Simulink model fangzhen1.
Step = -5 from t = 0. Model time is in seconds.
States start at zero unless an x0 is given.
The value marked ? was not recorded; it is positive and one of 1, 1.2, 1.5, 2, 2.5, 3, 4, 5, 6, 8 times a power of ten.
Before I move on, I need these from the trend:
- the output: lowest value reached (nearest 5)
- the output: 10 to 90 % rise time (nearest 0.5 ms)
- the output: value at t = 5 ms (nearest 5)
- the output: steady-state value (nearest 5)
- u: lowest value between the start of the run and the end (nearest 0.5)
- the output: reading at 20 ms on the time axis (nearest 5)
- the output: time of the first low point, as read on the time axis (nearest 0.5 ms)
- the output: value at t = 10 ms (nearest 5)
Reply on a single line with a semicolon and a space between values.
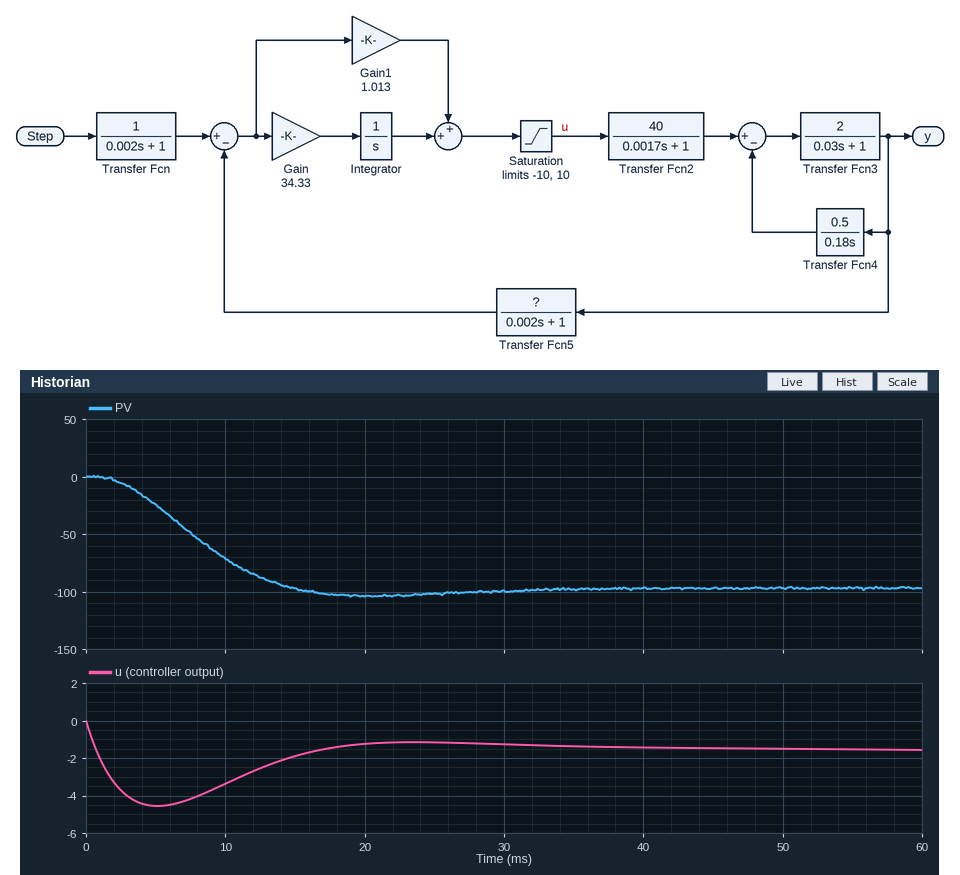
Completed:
-105; 9.0 ms; -25; -95; -4.5; -105; 20.5 ms; -70
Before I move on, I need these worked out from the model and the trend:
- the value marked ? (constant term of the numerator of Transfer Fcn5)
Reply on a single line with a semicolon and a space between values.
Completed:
0.05
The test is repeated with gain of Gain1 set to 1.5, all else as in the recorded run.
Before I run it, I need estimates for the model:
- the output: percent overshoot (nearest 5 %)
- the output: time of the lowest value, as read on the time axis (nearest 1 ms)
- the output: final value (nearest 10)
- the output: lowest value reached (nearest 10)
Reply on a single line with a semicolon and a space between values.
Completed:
15 %; 15 ms; -100; -110
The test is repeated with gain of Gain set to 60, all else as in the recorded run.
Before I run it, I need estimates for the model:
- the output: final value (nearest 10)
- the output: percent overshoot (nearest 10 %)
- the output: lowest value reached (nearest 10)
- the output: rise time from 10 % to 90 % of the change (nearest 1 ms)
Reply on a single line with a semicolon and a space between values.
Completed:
-100; 20 %; -120; 8 ms
